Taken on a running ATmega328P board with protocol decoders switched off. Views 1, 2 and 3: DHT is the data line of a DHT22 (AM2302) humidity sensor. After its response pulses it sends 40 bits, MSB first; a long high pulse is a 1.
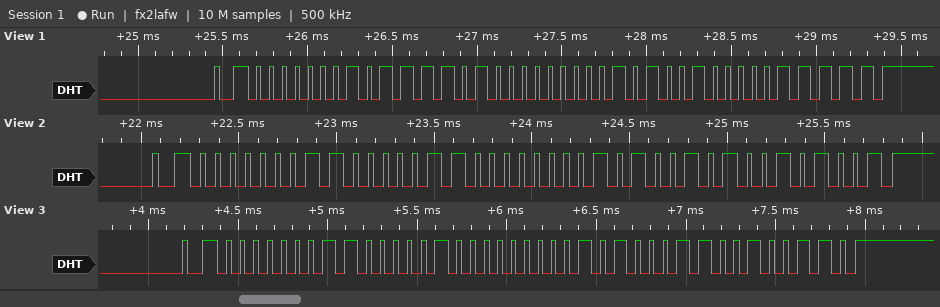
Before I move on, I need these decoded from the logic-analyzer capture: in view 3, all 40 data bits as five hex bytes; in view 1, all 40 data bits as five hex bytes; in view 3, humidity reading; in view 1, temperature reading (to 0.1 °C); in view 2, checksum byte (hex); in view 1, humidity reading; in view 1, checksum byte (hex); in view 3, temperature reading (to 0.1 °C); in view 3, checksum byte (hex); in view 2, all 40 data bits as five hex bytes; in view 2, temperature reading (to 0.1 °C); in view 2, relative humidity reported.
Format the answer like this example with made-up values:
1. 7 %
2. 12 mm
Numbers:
1. 01 82 00 A3 26
2. 01 7A 00 A4 1F
3. 38.6 %
4. 16.4 °C
5. 0x29
6. 37.8 %
7. 0x1F
8. 16.3 °C
9. 0x26
10. 01 83 00 A5 29
11. 16.5 °C
12. 38.7 %
